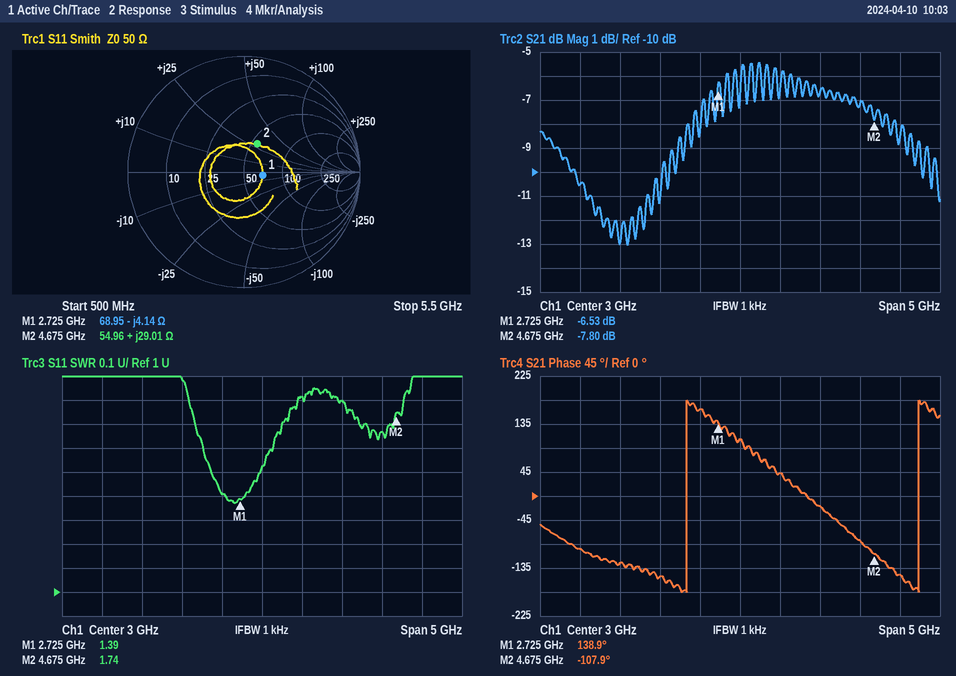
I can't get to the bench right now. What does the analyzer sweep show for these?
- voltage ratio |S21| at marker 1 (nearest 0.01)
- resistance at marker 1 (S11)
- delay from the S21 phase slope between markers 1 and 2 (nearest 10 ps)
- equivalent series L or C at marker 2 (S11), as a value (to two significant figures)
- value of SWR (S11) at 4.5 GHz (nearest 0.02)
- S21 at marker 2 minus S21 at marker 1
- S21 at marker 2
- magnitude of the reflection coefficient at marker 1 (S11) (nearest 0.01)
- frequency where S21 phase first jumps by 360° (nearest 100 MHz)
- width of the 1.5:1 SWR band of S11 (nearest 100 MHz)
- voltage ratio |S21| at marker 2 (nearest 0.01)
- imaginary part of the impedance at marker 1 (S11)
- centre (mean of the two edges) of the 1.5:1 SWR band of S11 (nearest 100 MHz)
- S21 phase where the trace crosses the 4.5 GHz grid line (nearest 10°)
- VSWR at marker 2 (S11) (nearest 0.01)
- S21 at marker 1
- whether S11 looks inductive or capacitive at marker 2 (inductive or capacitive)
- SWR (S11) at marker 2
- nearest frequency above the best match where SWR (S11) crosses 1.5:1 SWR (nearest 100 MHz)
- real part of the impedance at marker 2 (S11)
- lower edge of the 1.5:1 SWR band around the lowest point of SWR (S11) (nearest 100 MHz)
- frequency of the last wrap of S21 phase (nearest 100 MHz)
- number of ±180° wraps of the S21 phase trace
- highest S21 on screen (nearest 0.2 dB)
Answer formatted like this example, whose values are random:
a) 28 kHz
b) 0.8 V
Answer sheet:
a) 0.47
b) 68.95 Ω
c) 350 ps
d) 990 pH
e) 1.66
f) -1.27 dB
g) -7.80 dB
h) 0.16
i) 2.3 GHz
j) 600 MHz
k) 0.41
l) -4.14 Ω
m) 2.7 GHz
n) -80°
o) 1.74
p) -6.53 dB
q) inductive
r) 1.74
s) 3.0 GHz
t) 54.96 Ω
u) 2.4 GHz
v) 5.2 GHz
w) 2
x) -5.4 dB
